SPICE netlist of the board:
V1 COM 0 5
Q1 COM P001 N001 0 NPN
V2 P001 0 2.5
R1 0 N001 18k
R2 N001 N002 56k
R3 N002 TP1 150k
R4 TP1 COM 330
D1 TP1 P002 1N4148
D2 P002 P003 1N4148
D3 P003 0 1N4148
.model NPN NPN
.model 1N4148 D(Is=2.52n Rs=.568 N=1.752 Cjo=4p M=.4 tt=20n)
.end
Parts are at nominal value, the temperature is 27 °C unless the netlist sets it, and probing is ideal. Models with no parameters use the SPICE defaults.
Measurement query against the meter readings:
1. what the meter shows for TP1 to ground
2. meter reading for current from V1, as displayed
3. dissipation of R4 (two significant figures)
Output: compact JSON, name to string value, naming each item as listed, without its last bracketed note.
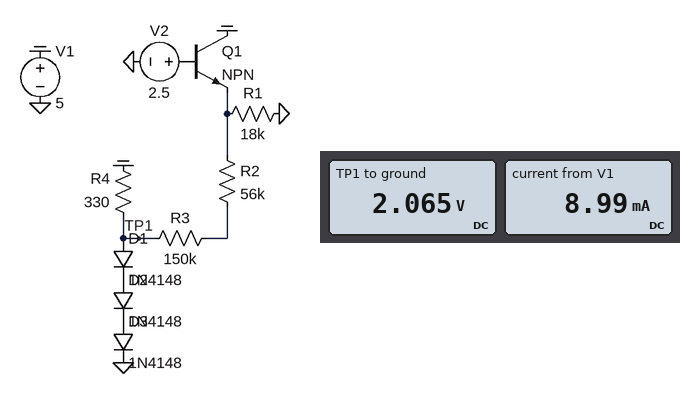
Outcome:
{"what the meter shows for TP1 to ground": "2.065 V", "meter reading for current from V1, as displayed": "8.99 mA", "dissipation of R4": "26 mW"}
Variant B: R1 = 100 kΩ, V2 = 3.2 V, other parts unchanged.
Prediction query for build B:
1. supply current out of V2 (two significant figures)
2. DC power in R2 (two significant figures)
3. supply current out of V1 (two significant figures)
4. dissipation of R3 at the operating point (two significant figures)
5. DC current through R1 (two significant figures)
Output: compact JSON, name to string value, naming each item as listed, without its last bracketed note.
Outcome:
{"supply current out of V2": "270 nA", "DC power in R2": "270 nW", "supply current out of V1": "8.9 mA", "dissipation of R3 at the operating point": "730 nW", "DC current through R1": "25 µA"}
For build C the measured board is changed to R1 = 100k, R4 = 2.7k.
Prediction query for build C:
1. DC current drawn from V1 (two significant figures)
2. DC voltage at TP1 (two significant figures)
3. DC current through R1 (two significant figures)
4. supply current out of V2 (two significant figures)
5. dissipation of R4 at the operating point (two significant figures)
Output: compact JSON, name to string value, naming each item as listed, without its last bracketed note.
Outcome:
{"DC current drawn from V1": "1.2 mA", "DC voltage at TP1": "1.8 V", "DC current through R1": "18 µA", "supply current out of V2": "180 nA", "dissipation of R4 at the operating point": "3.8 mW"}
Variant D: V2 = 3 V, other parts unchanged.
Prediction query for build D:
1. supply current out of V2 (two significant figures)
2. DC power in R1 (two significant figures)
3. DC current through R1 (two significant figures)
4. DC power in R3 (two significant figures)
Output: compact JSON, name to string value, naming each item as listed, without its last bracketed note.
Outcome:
{"supply current out of V2": "1.3 µA", "DC power in R1": "290 µW", "DC current through R1": "130 µA", "DC power in R3": "160 nW"}
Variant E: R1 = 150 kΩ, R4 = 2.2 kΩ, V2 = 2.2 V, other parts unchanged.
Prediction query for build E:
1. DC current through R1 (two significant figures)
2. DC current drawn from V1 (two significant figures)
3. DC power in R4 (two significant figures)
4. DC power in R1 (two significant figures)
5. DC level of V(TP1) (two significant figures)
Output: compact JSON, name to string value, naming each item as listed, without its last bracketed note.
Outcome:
{"DC current through R1": "10 µA", "DC current drawn from V1": "1.5 mA", "DC power in R4": "4.6 mW", "DC power in R1": "16 µW", "DC level of V(TP1)": "1.8 V"}
